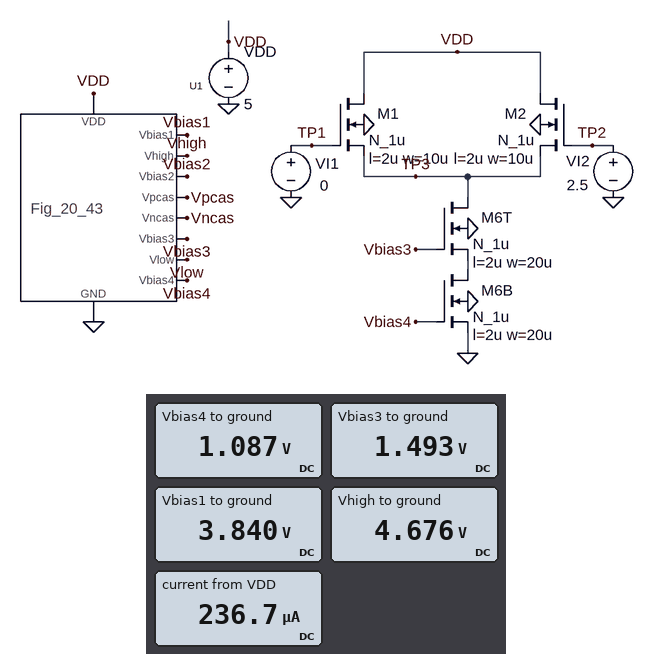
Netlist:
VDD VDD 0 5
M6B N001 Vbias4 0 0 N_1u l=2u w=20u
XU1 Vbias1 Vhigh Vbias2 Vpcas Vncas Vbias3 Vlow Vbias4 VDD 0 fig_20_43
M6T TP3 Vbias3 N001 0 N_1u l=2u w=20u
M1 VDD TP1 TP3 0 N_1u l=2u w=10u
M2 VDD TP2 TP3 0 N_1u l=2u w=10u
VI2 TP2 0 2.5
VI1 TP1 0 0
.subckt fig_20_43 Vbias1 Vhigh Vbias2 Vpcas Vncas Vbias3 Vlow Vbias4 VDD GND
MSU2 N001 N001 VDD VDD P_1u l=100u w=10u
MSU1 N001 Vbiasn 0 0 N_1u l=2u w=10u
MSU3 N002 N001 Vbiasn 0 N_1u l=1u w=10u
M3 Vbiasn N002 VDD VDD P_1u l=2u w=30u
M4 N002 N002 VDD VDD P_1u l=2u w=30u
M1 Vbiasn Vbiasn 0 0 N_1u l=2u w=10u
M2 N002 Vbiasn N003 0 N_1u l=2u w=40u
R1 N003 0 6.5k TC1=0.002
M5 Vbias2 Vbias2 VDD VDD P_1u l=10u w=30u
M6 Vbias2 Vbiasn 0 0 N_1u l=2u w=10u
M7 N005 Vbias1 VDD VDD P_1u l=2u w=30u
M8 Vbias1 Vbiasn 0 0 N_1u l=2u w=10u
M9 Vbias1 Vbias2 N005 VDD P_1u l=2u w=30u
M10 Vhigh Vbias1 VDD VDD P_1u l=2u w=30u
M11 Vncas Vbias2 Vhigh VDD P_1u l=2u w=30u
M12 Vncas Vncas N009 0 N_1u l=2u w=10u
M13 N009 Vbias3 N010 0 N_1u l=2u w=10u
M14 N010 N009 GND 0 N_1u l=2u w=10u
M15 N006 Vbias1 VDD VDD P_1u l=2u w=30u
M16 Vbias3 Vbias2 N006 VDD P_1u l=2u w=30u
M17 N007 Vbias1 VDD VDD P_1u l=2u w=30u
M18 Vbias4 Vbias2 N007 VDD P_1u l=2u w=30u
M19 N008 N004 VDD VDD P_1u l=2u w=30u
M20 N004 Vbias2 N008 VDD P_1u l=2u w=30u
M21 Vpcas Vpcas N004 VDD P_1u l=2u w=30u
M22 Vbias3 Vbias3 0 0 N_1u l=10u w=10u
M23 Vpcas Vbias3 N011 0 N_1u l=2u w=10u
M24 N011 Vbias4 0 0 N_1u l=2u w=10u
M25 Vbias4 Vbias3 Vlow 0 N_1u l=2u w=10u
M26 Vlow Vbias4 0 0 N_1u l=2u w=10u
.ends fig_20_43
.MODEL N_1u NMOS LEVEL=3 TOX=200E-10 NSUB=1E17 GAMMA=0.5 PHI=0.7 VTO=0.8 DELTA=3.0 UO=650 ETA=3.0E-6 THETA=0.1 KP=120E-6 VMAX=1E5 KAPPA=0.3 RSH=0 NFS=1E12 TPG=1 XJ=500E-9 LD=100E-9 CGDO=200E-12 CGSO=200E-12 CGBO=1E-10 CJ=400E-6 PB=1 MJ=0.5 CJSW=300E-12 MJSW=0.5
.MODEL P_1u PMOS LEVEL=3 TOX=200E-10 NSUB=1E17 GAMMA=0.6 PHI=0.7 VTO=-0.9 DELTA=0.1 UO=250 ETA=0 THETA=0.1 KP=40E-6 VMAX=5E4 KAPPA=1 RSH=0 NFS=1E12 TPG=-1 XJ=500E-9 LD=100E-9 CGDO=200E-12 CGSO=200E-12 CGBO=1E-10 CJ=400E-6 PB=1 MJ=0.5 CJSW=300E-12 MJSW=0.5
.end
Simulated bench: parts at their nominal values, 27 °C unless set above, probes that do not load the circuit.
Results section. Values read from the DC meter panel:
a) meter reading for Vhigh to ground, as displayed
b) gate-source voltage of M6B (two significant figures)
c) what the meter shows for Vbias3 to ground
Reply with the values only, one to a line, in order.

4.676 V
1.1 V
1.493 V
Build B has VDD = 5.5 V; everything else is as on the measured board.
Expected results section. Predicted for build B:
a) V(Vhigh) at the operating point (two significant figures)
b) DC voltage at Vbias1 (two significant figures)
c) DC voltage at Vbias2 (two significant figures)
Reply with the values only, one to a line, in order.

5.2 V
4.3 V
3.9 V
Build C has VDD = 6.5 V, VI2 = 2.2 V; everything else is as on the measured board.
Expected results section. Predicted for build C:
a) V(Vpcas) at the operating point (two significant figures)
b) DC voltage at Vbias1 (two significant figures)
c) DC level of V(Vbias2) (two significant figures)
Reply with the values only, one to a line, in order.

3.9 V
5.3 V
4.9 V
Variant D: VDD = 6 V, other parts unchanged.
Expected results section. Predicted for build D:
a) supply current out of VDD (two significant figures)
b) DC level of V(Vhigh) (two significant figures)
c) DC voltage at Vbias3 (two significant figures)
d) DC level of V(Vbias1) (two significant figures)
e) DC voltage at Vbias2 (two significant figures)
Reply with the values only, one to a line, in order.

250 µA
5.7 V
1.5 V
4.8 V
4.4 V
